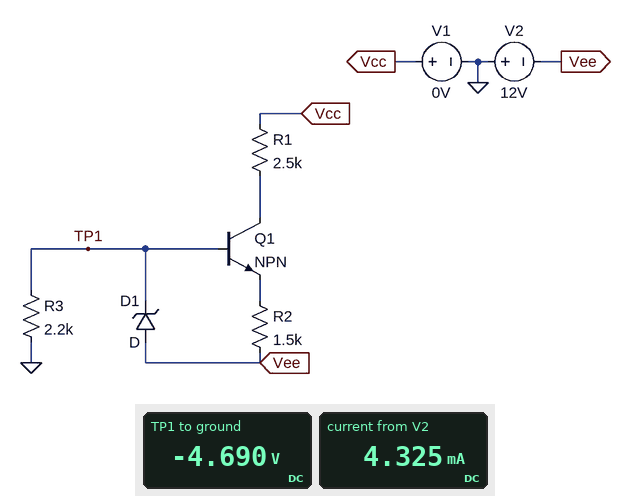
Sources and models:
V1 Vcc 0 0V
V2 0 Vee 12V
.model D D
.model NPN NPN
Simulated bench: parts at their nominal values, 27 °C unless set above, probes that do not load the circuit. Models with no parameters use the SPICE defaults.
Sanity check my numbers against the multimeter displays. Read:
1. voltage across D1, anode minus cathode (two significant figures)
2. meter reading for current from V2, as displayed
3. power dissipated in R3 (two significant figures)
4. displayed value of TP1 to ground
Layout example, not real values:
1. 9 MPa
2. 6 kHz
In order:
1. -7.3 V
2. 4.325 mA
3. 10 mW
4. -4.690 V
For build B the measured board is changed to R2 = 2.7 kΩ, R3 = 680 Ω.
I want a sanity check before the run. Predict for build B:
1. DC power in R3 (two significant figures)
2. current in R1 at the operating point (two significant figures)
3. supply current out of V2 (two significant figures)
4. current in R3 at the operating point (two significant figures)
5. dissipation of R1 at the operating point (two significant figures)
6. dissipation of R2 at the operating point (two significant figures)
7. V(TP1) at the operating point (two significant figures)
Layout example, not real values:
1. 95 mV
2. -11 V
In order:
1. 4.3 mW
2. 1.0 mA
3. 3.5 mA
4. 2.5 mA
5. 2.5 mW
6. 33 mW
7. -1.7 V
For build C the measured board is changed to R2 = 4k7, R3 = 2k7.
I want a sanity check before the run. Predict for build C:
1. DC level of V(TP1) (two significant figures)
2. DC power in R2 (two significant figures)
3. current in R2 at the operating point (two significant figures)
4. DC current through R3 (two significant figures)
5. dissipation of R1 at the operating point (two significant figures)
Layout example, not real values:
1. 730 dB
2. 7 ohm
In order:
1. -2.1 V
2. 18 mW
3. 1.9 mA
4. 780 µA
5. 3.3 mW
